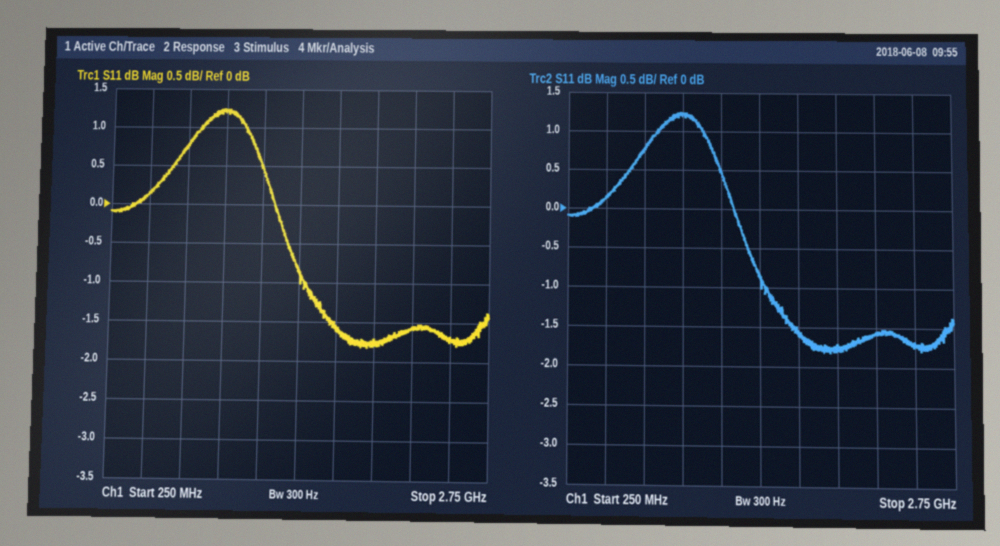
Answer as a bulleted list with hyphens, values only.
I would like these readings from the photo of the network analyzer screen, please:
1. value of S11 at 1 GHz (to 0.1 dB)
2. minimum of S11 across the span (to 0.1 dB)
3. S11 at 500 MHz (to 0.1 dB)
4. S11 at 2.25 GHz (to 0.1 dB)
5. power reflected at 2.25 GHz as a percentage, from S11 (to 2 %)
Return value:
- 1.2 dB
- -1.8 dB
- 0.1 dB
- -1.6 dB
- 70 %
